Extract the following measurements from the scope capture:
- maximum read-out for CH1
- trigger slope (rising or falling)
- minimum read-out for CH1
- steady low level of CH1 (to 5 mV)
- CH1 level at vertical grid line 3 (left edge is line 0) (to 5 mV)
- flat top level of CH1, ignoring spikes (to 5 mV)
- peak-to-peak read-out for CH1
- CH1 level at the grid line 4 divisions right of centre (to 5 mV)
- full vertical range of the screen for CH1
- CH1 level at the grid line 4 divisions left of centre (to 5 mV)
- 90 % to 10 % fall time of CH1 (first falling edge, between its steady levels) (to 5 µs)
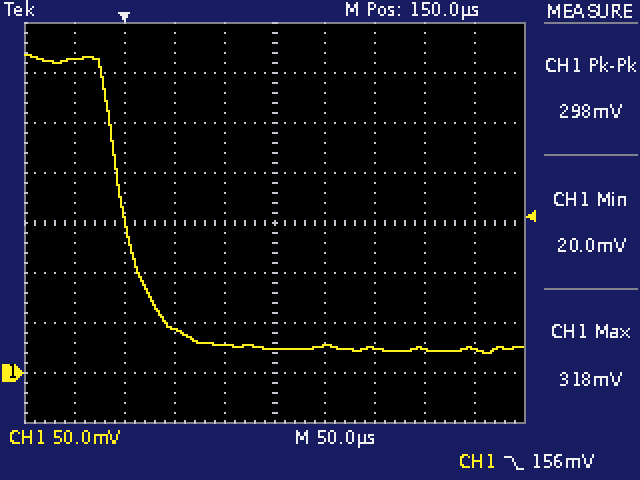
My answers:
318 mV
falling
20.0 mV
25 mV
45 mV
315 mV
298 mV
25 mV
400 mV
315 mV
60 µs
